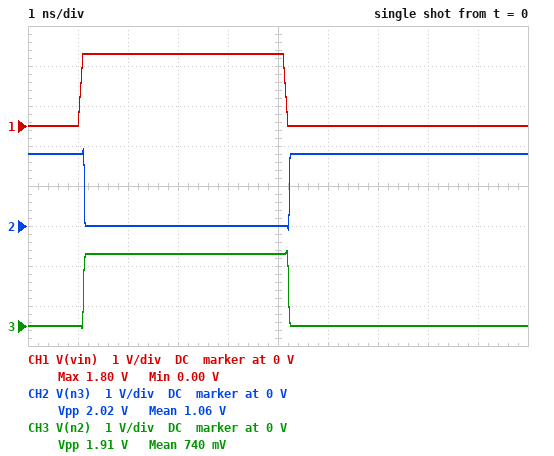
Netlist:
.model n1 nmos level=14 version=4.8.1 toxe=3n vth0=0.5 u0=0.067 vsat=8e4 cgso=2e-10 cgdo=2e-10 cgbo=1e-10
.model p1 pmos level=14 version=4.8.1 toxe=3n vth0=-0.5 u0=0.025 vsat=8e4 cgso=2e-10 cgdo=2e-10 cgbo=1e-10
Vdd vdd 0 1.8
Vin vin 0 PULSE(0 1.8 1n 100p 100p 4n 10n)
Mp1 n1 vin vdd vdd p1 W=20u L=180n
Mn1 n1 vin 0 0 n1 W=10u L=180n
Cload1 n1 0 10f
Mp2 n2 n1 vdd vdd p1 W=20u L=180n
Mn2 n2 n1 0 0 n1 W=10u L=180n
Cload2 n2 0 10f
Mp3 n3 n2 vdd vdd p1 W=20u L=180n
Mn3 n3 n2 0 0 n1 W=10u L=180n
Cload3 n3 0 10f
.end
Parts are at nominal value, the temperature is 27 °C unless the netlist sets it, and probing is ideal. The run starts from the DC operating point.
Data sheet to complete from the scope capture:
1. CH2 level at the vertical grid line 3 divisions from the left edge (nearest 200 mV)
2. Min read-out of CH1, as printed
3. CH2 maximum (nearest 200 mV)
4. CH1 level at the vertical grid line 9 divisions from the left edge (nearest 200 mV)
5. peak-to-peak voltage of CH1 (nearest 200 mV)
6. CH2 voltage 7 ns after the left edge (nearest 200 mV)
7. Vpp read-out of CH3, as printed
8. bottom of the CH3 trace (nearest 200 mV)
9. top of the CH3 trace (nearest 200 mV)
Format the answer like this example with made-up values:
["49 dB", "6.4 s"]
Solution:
["0 V", "0.00 V", "2.0 V", "0 V", "1.8 V", "1.8 V", "1.91 V", "0 V", "1.8 V"]
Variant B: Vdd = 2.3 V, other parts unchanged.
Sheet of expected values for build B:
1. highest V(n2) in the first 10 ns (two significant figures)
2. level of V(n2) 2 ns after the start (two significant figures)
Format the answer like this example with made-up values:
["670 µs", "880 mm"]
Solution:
["2.4 V", "2.3 V"]
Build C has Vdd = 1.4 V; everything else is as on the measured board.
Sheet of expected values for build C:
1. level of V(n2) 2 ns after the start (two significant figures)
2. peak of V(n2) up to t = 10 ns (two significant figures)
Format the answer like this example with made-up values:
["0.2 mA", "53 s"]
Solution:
["1.4 V", "1.5 V"]
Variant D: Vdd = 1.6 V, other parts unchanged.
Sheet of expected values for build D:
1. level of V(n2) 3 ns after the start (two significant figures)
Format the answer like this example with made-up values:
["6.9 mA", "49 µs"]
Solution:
["1.6 V"]
